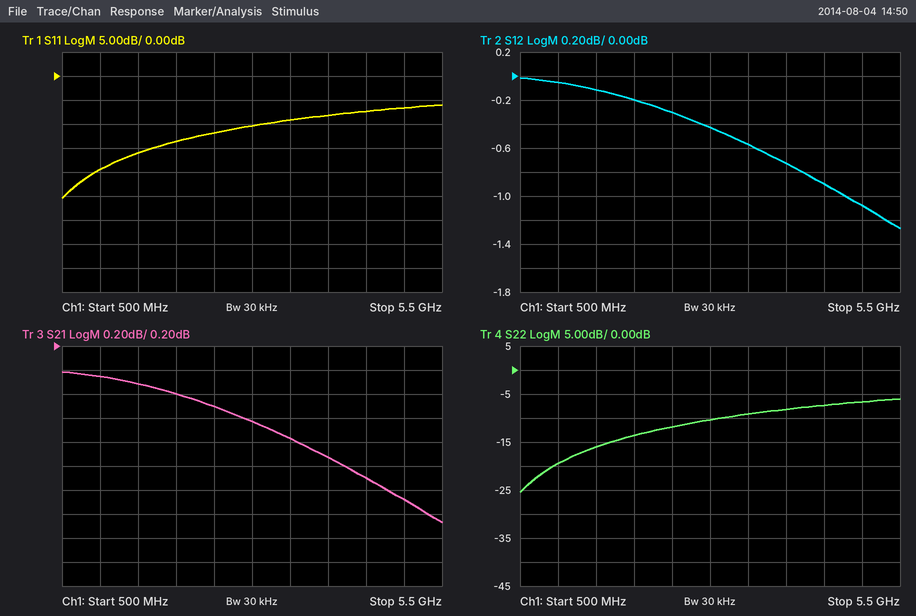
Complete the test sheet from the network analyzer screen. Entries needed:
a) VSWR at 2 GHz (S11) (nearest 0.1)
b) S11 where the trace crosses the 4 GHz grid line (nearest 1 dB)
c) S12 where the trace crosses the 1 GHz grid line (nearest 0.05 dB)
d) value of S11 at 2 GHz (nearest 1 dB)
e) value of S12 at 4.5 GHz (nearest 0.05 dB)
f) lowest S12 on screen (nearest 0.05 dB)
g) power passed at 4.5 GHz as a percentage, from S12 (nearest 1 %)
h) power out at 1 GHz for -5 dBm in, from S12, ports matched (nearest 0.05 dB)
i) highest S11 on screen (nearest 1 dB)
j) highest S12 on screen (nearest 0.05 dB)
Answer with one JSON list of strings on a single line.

["1.5", "-8 dB", "-0.05 dB", "-14 dB", "-0.90 dB", "-1.25 dB", "81 %", "-5.05 dBm", "-6 dB", "0.00 dB"]
